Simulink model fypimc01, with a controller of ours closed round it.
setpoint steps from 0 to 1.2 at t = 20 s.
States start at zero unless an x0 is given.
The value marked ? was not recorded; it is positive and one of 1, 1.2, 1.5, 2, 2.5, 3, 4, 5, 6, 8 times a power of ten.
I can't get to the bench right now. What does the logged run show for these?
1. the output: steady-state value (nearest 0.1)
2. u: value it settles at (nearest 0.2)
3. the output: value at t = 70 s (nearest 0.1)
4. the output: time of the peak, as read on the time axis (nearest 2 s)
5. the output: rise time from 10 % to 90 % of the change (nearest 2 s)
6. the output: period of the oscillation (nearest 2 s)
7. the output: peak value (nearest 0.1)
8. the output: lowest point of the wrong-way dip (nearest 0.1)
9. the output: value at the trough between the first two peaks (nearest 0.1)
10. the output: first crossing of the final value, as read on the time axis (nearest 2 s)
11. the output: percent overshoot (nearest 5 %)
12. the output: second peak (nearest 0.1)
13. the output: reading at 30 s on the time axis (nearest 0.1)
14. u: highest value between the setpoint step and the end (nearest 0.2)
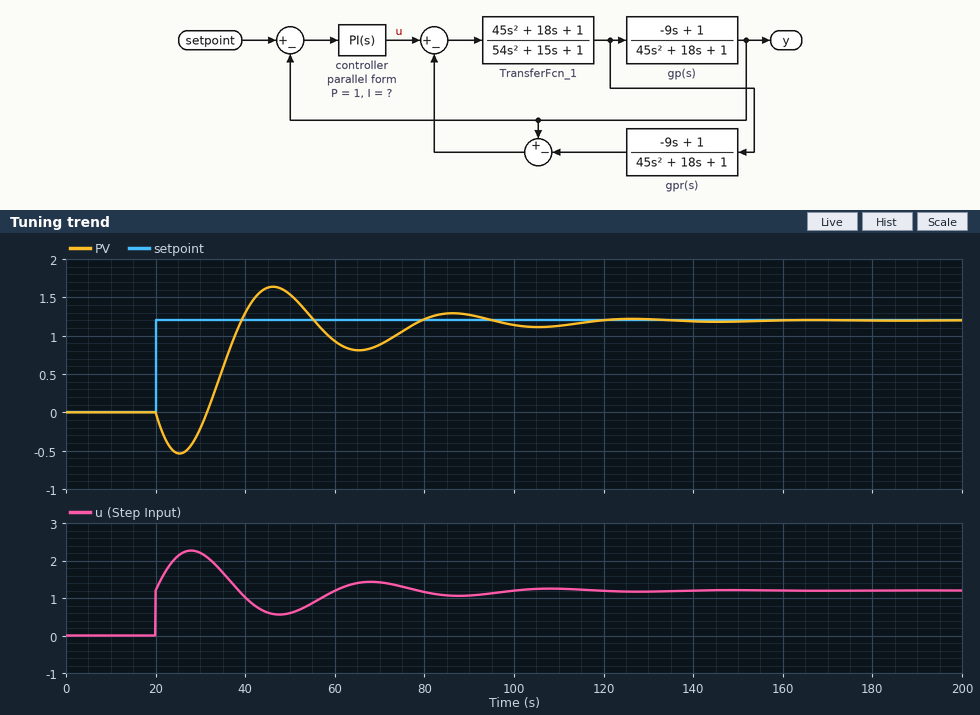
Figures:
1.2
1.2
0.9
46 s
6 s
40 s
1.6
-0.5
0.8
40 s
35 %
1.3
-0.2
2.2
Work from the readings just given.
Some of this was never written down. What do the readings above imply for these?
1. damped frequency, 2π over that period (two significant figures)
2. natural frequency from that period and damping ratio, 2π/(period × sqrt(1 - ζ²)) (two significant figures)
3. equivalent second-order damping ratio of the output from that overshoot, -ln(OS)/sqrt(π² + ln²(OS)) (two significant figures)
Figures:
0.16 rad/s
0.17 rad/s
0.32
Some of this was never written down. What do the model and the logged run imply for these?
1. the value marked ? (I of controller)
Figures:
0.05
